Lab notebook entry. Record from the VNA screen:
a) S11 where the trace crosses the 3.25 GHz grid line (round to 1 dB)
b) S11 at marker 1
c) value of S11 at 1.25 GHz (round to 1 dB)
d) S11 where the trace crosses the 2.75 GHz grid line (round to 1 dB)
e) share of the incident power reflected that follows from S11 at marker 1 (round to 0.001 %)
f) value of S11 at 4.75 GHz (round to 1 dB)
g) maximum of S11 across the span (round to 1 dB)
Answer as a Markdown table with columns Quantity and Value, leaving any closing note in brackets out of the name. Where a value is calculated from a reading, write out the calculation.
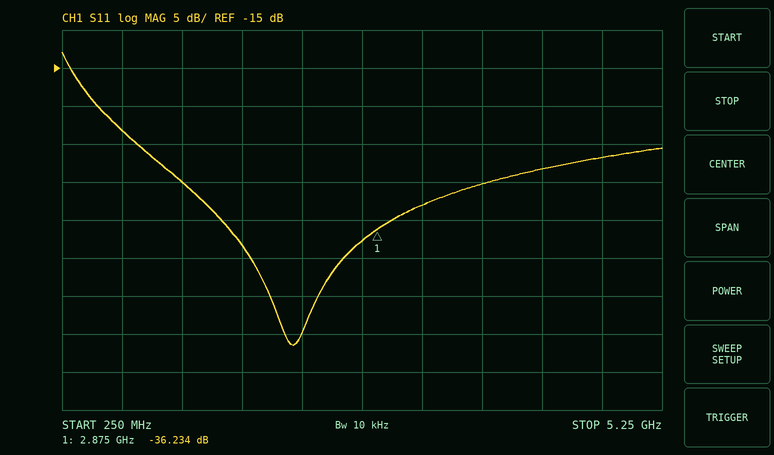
| Quantity | Value |
|---|---|
| S11 where the trace crosses the 3.25 GHz grid line | -33 dB |
| S11 at marker 1 | -36.234 dB |
| value of S11 at 1.25 GHz | -30 dB |
| S11 where the trace crosses the 2.75 GHz grid line | -38 dB |
| share of the incident power reflected that follows from S11 at marker 1 | 10^(-36.234/10) ≈ 0.024 % |
| value of S11 at 4.75 GHz | -27 dB |
| maximum of S11 across the span | -13 dB |
